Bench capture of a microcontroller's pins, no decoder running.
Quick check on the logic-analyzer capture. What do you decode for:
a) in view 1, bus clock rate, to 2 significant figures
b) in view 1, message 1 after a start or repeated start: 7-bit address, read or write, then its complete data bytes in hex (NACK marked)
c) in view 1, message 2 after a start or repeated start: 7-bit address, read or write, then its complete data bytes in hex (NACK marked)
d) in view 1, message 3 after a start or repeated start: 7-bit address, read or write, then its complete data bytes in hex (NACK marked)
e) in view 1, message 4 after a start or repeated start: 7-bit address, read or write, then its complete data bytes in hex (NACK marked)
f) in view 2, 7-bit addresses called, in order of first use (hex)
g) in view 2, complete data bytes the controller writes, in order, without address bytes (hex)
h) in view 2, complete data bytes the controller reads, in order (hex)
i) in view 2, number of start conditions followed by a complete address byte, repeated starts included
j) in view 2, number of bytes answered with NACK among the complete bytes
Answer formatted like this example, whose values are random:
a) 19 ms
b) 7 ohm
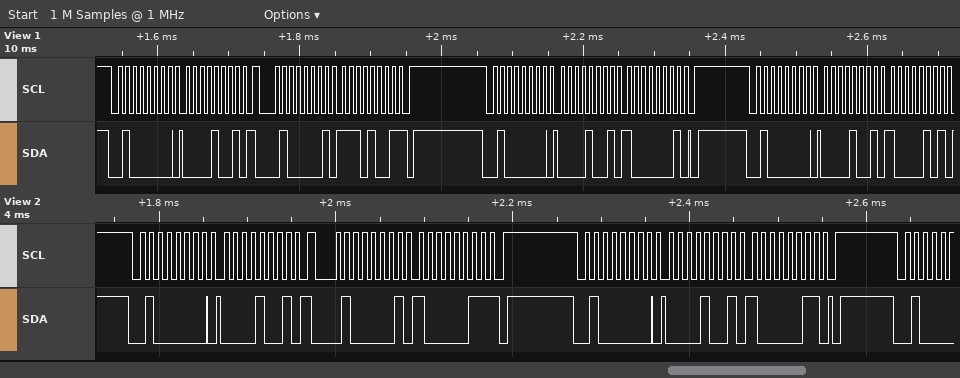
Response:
a) 100 kHz
b) 0x20 write: 09
c) 0x20 read: E9 NACK
d) 0x20 write: 09 81
e) 0x20 write: 09 85
f) 0x20
g) 09 09 83
h) 83
i) 3
j) 1
